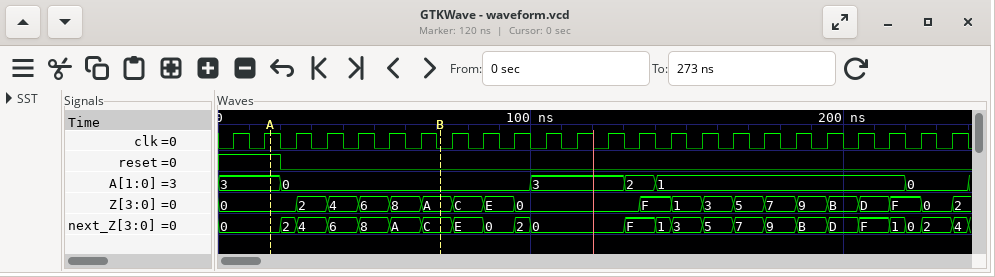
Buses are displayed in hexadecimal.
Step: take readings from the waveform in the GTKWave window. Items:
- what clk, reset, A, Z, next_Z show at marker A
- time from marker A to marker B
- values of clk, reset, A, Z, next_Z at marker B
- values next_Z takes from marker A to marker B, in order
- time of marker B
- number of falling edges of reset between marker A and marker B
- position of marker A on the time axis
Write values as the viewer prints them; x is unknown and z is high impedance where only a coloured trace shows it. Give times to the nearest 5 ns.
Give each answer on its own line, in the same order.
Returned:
clk=1, reset=1, A=3, Z=0, next_Z=0
55 ns
clk=0, reset=0, A=0, Z=A, next_Z=C
0, 2, 4, 6, 8, A, C
70 ns
1
15 ns
